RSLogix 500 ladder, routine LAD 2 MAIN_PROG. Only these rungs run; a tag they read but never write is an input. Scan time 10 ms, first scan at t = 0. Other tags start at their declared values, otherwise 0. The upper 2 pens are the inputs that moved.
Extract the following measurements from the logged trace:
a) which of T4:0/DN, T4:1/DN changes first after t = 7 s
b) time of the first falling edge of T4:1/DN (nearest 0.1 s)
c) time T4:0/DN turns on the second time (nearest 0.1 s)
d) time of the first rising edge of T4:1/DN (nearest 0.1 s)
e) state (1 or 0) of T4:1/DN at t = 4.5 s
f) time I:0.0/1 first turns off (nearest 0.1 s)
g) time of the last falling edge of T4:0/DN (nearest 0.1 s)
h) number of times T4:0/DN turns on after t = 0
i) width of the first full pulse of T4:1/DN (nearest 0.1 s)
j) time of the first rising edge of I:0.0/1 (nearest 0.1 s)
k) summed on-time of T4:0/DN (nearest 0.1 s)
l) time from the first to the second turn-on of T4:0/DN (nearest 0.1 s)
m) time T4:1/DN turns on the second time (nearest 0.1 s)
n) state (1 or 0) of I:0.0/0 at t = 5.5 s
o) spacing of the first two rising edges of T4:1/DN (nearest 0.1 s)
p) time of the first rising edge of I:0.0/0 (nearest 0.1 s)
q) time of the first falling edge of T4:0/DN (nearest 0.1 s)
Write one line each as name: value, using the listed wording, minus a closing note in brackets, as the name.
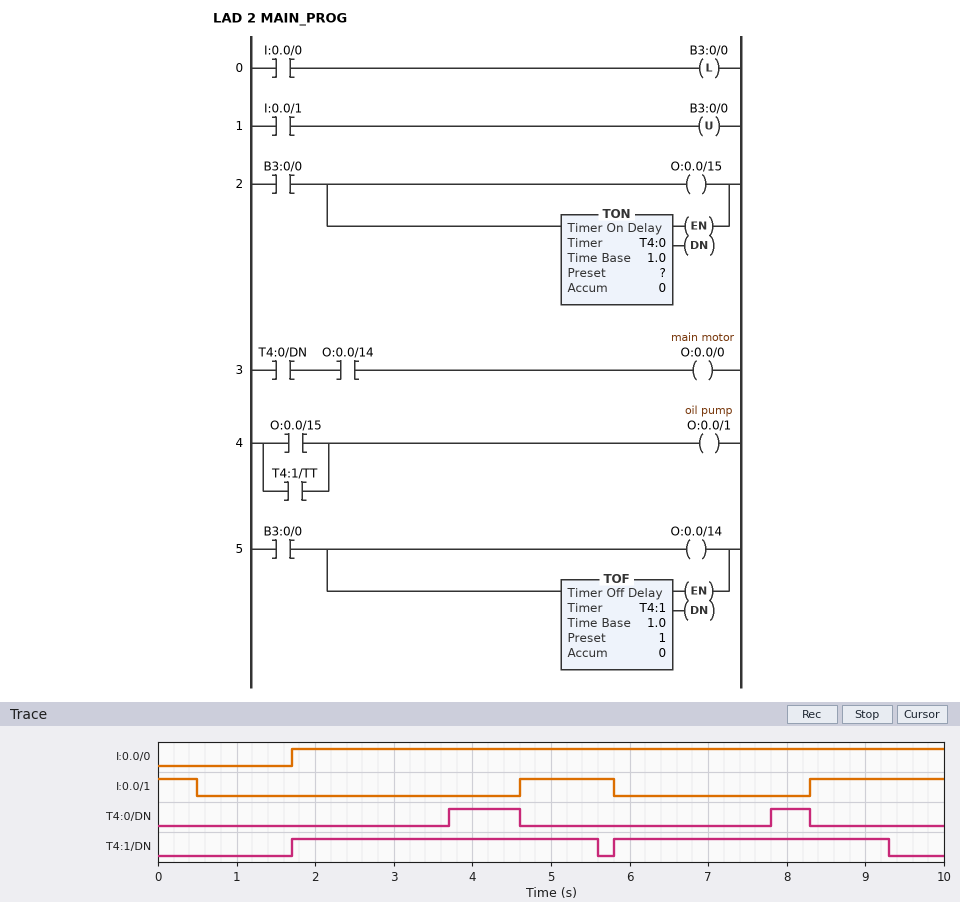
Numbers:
which of T4:0/DN, T4:1/DN changes first after t = 7 s: T4:0/DN
time of the first falling edge of T4:1/DN: 5.6 s
time T4:0/DN turns on the second time: 7.8 s
time of the first rising edge of T4:1/DN: 1.7 s
state (1 or 0) of T4:1/DN at t = 4.5 s: 1
time I:0.0/1 first turns off: 0.5 s
time of the last falling edge of T4:0/DN: 8.3 s
number of times T4:0/DN turns on after t = 0: 2
width of the first full pulse of T4:1/DN: 3.9 s
time of the first rising edge of I:0.0/1: 4.6 s
summed on-time of T4:0/DN: 1.4 s
time from the first to the second turn-on of T4:0/DN: 4.1 s
time T4:1/DN turns on the second time: 5.8 s
state (1 or 0) of I:0.0/0 at t = 5.5 s: 1
spacing of the first two rising edges of T4:1/DN: 4.1 s
time of the first rising edge of I:0.0/0: 1.7 s
time of the first falling edge of T4:0/DN: 4.6 s
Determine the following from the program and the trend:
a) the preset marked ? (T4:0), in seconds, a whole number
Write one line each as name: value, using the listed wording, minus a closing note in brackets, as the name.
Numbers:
the preset marked ? (T4:0), in seconds, a whole number: 2 s
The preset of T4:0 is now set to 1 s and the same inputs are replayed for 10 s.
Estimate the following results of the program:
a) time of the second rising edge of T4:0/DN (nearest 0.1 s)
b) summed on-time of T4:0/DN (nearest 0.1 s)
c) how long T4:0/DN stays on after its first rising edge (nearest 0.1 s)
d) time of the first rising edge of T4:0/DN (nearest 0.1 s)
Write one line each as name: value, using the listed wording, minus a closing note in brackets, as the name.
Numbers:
time of the second rising edge of T4:0/DN: 6.8 s
summed on-time of T4:0/DN: 3.4 s
how long T4:0/DN stays on after its first rising edge: 1.9 s
time of the first rising edge of T4:0/DN: 2.7 s
